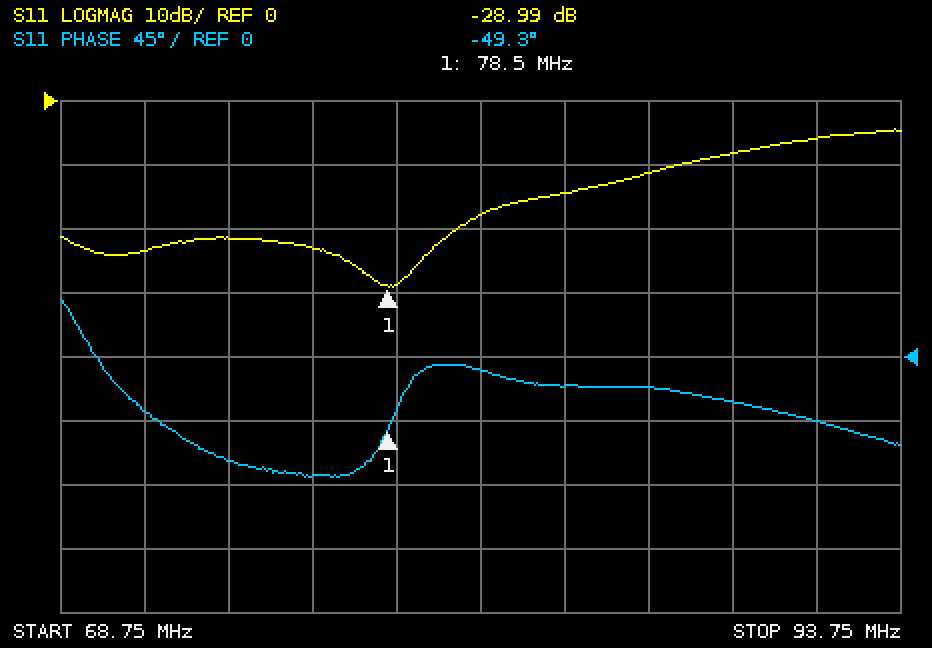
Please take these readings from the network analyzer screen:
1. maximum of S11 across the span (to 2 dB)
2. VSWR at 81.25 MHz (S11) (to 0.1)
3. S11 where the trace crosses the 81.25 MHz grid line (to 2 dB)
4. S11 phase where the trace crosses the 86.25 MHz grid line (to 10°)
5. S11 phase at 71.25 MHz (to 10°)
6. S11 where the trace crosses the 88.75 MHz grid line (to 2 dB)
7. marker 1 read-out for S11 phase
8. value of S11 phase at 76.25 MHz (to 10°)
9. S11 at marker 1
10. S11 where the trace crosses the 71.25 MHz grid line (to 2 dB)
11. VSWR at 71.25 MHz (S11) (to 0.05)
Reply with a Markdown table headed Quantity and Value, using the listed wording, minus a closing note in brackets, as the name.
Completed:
| Quantity | Value |
|---|---|
| maximum of S11 across the span | -4 dB |
| VSWR at 81.25 MHz (S11) | 1.3 |
| S11 where the trace crosses the 81.25 MHz grid line | -18 dB |
| S11 phase where the trace crosses the 86.25 MHz grid line | -20° |
| S11 phase at 71.25 MHz | -40° |
| S11 where the trace crosses the 88.75 MHz grid line | -8 dB |
| marker 1 read-out for S11 phase | -49.3° |
| value of S11 phase at 76.25 MHz | -80° |
| S11 at marker 1 | -28.99 dB |
| S11 where the trace crosses the 71.25 MHz grid line | -24 dB |
| VSWR at 71.25 MHz (S11) | 1.15 |
